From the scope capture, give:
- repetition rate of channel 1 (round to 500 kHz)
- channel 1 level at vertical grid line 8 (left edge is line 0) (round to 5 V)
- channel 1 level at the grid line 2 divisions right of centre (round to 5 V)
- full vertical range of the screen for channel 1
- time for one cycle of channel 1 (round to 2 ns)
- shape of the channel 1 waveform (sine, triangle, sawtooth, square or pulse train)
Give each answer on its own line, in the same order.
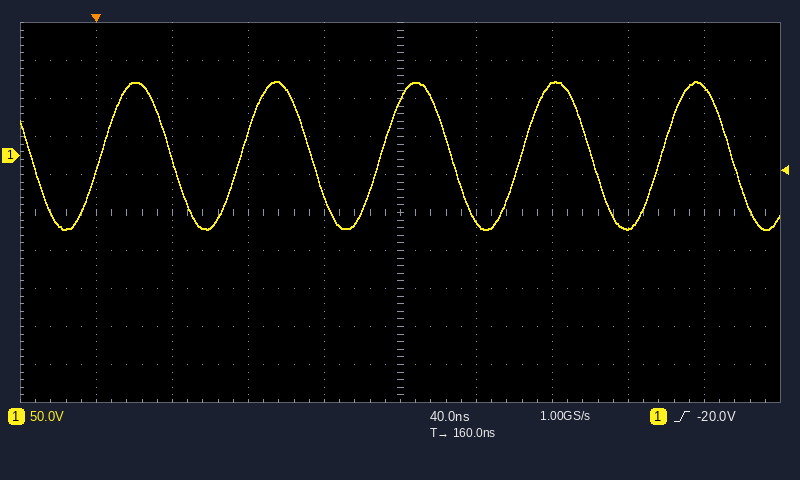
13.5 MHz
-95 V
95 V
500 V
74 ns
sine
